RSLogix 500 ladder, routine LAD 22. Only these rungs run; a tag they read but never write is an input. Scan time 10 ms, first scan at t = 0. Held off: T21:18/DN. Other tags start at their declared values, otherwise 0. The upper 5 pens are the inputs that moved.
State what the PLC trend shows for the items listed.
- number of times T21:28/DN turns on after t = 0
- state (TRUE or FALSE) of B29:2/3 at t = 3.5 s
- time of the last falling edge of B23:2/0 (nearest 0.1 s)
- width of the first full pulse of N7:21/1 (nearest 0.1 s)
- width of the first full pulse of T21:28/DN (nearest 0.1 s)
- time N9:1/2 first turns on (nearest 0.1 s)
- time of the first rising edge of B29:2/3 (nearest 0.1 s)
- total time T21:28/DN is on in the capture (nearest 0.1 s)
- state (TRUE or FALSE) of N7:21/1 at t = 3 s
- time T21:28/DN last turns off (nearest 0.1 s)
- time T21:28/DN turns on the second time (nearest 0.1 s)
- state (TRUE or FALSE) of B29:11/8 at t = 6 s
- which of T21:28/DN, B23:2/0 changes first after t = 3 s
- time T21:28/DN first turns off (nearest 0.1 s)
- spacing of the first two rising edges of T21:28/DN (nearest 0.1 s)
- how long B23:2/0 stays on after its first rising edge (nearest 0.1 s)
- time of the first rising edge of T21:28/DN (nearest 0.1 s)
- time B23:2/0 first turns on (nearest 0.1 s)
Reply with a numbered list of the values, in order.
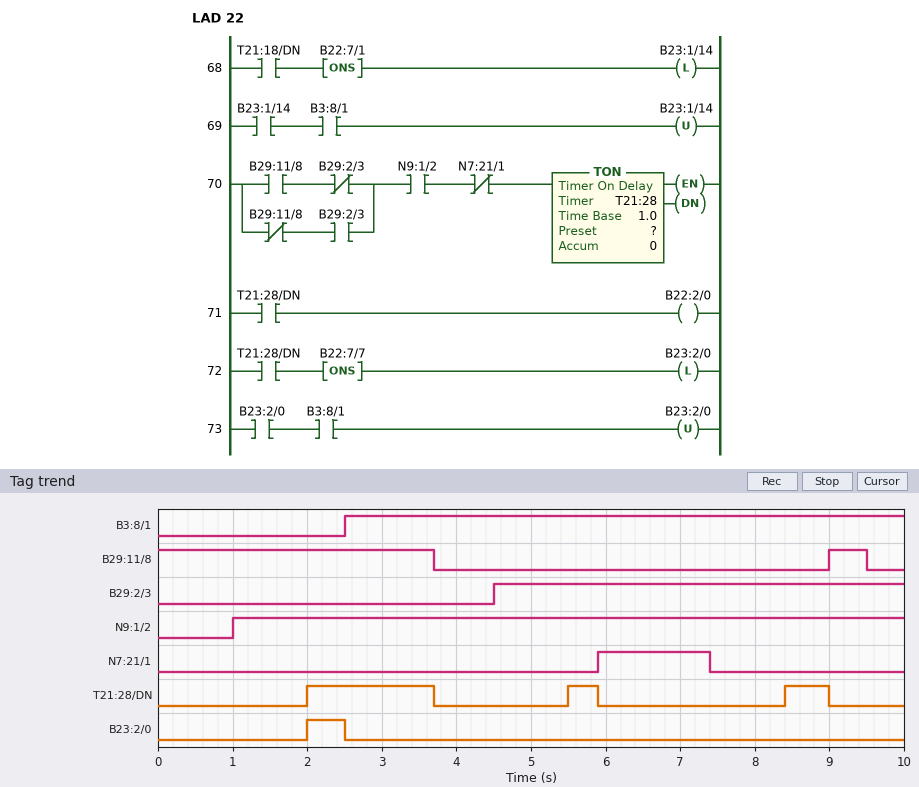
1. 3
2. FALSE
3. 2.5 s
4. 1.5 s
5. 1.7 s
6. 1.0 s
7. 4.5 s
8. 2.7 s
9. FALSE
10. 9.0 s
11. 5.5 s
12. FALSE
13. T21:28/DN
14. 3.7 s
15. 3.5 s
16. 0.5 s
17. 2.0 s
18. 2.0 s
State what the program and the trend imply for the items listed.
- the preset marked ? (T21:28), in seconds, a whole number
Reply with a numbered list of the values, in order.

1. 1 s
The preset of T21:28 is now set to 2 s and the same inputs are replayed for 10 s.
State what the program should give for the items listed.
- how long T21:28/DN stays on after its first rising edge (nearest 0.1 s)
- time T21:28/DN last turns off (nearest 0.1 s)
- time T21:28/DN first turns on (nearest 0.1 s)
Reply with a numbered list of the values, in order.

1. 0.7 s
2. 3.7 s
3. 3.0 s
